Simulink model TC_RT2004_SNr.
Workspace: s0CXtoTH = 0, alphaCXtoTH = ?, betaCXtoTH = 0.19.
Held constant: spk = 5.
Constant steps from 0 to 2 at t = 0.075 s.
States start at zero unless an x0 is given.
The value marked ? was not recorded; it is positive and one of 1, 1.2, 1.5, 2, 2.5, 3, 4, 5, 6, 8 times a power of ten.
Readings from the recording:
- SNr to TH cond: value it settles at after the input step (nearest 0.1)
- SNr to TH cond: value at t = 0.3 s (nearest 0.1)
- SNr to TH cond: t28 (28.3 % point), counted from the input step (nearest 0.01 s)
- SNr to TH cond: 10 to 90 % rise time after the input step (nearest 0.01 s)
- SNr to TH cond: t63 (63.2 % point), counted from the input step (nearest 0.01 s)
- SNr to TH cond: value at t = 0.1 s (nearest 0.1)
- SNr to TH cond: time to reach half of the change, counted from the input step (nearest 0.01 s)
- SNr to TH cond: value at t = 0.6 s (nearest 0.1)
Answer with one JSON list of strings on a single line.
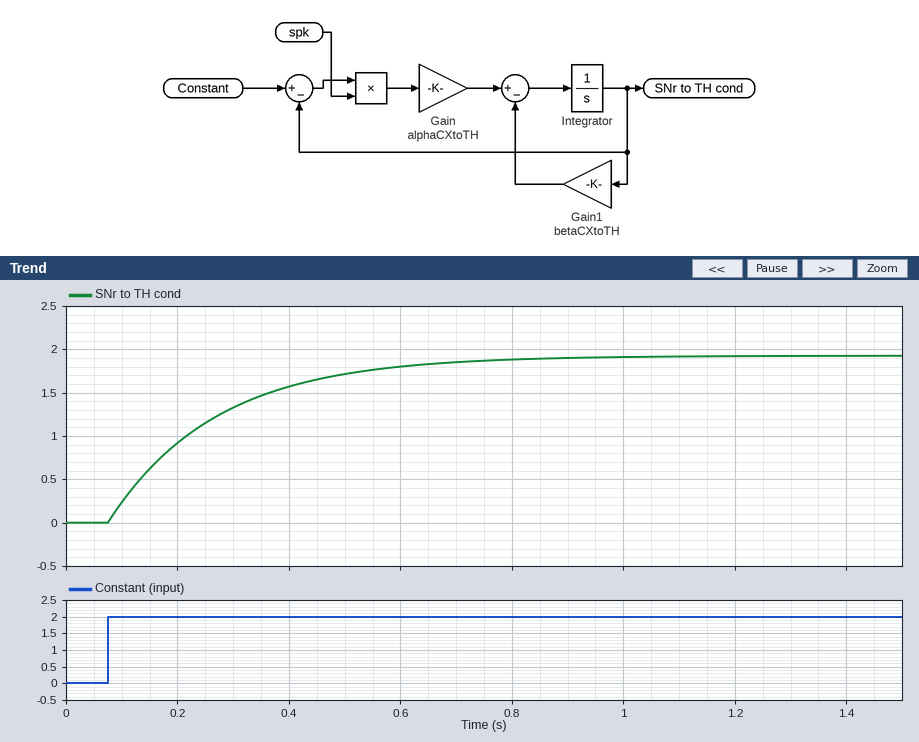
["1.9", "1.3", "0.06 s", "0.42 s", "0.19 s", "0.2", "0.13 s", "1.8"]
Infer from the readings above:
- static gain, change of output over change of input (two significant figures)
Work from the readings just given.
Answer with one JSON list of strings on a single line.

["0.95"]
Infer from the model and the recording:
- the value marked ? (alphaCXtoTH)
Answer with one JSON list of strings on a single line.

["1"]
